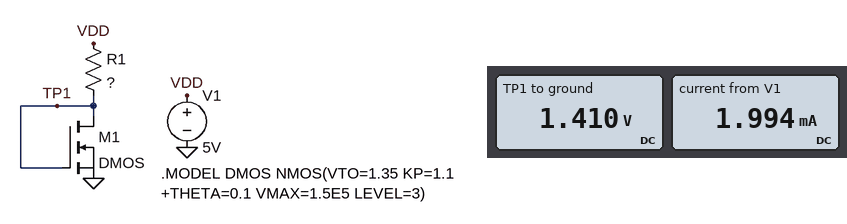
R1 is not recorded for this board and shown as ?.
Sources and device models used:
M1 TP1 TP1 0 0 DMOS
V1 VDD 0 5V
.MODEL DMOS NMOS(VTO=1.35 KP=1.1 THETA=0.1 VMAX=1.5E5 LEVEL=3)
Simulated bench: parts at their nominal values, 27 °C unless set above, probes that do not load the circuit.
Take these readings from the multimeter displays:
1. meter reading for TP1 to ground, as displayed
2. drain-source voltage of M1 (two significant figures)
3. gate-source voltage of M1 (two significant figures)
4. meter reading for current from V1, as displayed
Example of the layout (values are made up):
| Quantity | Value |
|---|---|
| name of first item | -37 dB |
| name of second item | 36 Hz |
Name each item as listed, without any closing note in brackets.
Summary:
| Quantity | Value |
|---|---|
| meter reading for TP1 to ground, as displayed | 1.410 V |
| drain-source voltage of M1 | 1.4 V |
| gate-source voltage of M1 | 1.4 V |
| meter reading for current from V1, as displayed | 1.994 mA |
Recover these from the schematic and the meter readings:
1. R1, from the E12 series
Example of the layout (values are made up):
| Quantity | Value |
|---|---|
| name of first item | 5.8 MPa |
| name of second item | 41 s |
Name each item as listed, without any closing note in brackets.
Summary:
| Quantity | Value |
|---|---|
| R1, from the E12 series | 1.8 kΩ |
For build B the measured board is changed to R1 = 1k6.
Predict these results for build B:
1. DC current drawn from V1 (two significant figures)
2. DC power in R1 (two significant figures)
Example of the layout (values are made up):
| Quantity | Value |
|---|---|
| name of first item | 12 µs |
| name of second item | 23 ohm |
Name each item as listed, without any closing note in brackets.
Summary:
| Quantity | Value |
|---|---|
| DC current drawn from V1 | 2.2 mA |
| DC power in R1 | 8.0 mW |
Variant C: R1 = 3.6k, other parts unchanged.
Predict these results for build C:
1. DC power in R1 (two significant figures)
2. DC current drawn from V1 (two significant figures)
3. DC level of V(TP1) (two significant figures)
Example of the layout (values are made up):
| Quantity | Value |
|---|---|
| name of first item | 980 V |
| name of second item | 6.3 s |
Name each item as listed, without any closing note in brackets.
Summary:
| Quantity | Value |
|---|---|
| DC power in R1 | 3.6 mW |
| DC current drawn from V1 | 1.0 mA |
| DC level of V(TP1) | 1.4 V |
